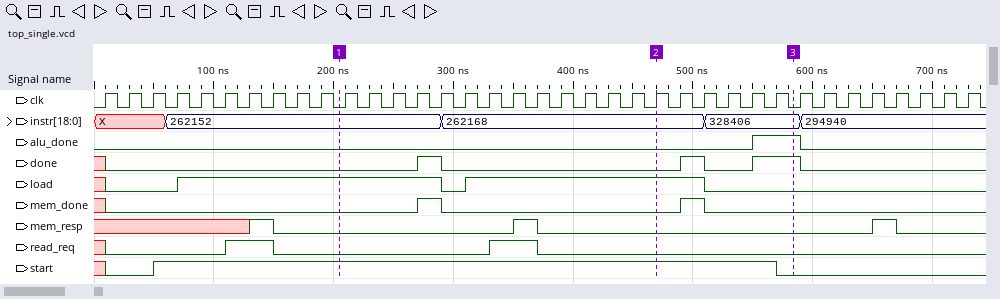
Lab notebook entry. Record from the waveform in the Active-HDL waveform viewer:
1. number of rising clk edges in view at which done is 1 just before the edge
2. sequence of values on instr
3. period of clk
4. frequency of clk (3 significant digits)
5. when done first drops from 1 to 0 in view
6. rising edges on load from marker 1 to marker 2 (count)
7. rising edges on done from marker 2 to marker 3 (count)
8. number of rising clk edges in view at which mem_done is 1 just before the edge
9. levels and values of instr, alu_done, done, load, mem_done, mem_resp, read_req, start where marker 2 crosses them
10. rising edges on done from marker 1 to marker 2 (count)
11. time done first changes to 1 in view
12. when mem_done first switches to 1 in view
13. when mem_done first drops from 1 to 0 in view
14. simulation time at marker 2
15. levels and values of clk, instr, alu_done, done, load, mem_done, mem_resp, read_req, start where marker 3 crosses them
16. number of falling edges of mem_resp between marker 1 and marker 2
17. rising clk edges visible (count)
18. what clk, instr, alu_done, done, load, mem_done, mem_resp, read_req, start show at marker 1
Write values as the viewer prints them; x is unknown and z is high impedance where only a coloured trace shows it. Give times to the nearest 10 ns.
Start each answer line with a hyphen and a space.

- 4
- X, 262152, 262168, 328406, 294940
- 20 ns
- 50.0 MHz
- 290 ns
- 1
- 2
- 2
- instr=262168, alu_done=0, done=0, load=1, mem_done=0, mem_resp=0, read_req=0, start=1
- 1
- 270 ns
- 270 ns
- 290 ns
- 470 ns
- clk=0, instr=328406, alu_done=1, done=1, load=0, mem_done=0, mem_resp=0, read_req=0, start=0
- 1
- 37
- clk=0, instr=262152, alu_done=0, done=0, load=1, mem_done=0, mem_resp=0, read_req=0, start=1
